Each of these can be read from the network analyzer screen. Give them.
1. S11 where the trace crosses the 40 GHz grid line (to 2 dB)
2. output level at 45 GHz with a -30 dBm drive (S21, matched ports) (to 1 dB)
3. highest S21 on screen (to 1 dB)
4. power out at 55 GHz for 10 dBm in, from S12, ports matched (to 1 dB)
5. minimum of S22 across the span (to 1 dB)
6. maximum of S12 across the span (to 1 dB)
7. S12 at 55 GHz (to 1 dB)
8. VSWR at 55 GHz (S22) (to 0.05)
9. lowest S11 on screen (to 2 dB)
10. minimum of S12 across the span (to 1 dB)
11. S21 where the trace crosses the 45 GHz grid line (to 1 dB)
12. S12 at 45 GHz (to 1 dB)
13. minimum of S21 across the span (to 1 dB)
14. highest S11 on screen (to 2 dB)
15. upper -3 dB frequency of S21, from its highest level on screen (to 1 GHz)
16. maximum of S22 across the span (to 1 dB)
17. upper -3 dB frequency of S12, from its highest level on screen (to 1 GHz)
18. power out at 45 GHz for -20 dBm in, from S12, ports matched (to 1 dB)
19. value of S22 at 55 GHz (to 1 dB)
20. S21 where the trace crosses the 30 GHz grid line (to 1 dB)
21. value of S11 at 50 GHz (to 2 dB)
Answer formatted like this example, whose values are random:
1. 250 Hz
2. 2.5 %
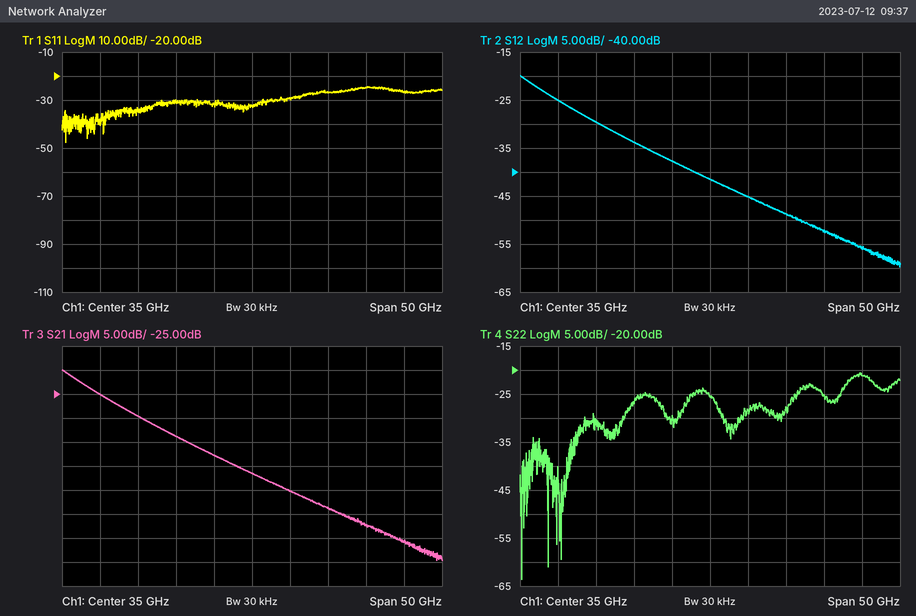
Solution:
1. -30 dB
2. -79 dBm
3. -20 dB
4. -46 dBm
5. -64 dB
6. -20 dB
7. -56 dB
8. 1.20
9. -48 dB
10. -60 dB
11. -49 dB
12. -49 dB
13. -60 dB
14. -24 dB
15. 13 GHz
16. -21 dB
17. 13 GHz
18. -69 dBm
19. -21 dB
20. -38 dB
21. -24 dB
